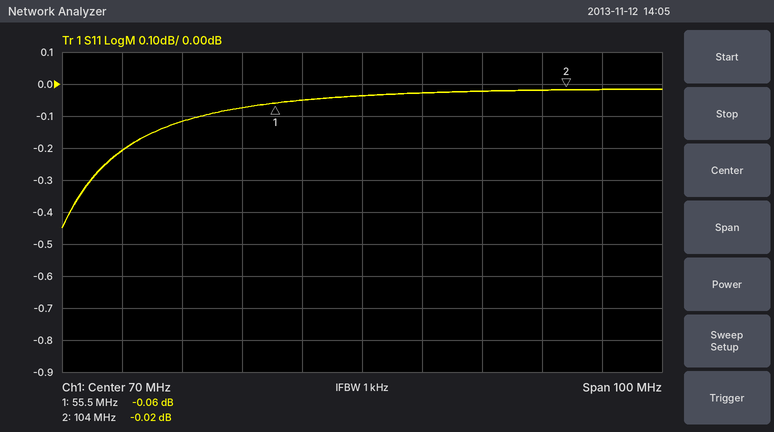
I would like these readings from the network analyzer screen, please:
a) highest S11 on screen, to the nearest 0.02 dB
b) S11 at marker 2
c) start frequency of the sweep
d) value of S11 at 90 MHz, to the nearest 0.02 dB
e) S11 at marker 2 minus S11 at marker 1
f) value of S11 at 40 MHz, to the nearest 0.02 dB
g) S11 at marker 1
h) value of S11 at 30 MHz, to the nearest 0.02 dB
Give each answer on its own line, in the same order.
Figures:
-0.02 dB
-0.02 dB
20 MHz
-0.02 dB
0.04 dB
-0.12 dB
-0.06 dB
-0.20 dB
